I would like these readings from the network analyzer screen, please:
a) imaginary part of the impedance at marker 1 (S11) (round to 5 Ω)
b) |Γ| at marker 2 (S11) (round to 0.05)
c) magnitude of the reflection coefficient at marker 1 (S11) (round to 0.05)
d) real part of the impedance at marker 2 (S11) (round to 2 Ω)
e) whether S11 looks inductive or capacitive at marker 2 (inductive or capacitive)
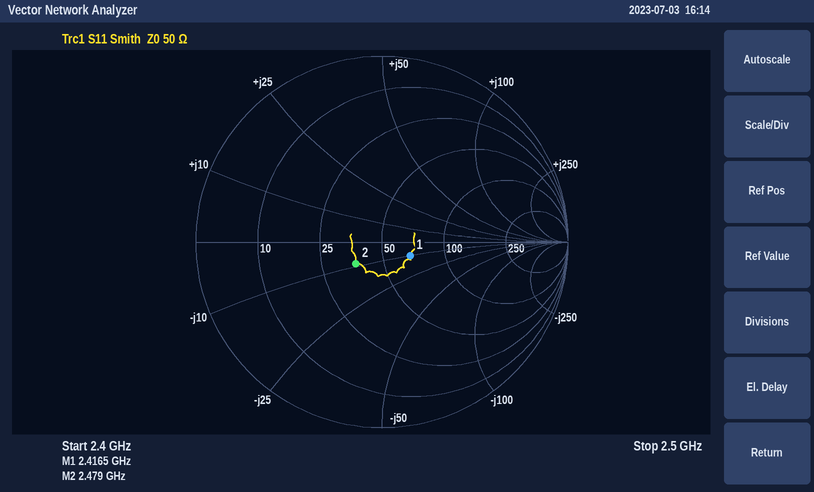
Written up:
-10 Ω
0.20
0.15
36 Ω
capacitive
